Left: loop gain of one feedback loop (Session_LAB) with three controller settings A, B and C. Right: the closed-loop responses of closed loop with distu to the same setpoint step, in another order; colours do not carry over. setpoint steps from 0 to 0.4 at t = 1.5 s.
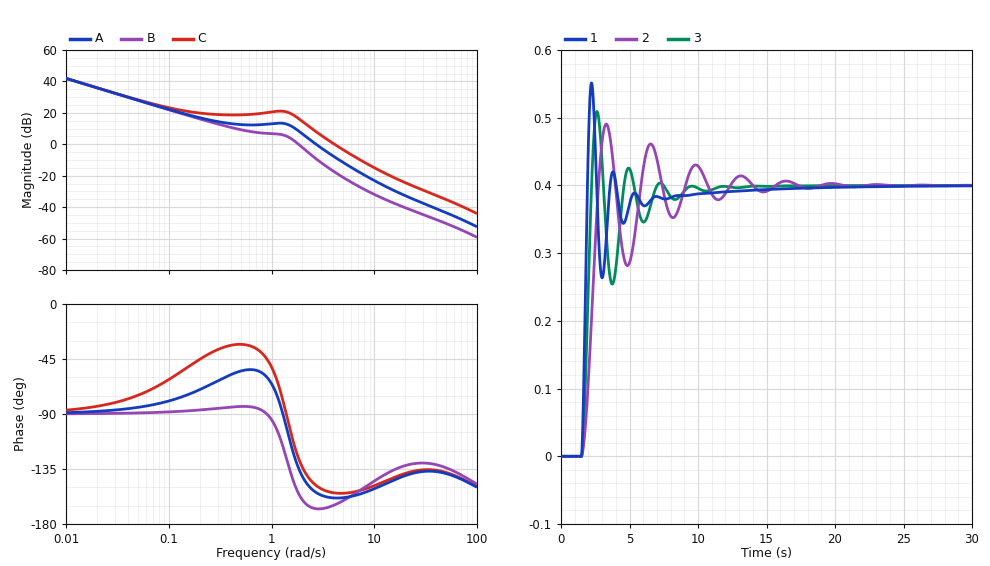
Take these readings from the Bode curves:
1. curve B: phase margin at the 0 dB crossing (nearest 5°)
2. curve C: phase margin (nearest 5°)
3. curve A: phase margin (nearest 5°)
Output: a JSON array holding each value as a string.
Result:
["25°", "25°", "25°"]
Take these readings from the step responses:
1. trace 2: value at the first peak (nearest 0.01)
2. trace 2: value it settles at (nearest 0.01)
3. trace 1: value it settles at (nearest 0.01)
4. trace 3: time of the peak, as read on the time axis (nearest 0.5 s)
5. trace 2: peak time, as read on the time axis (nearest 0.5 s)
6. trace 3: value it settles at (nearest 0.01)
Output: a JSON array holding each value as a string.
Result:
["0.49", "0.40", "0.40", "2.5 s", "3.5 s", "0.40"]
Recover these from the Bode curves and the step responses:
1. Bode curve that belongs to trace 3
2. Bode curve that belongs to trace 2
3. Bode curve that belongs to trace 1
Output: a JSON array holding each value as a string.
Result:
["A", "B", "C"]
